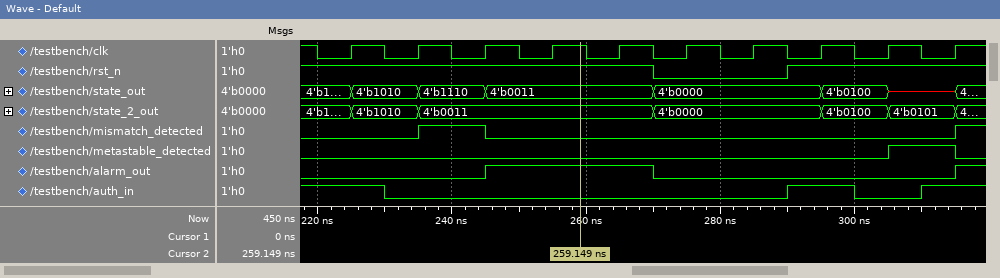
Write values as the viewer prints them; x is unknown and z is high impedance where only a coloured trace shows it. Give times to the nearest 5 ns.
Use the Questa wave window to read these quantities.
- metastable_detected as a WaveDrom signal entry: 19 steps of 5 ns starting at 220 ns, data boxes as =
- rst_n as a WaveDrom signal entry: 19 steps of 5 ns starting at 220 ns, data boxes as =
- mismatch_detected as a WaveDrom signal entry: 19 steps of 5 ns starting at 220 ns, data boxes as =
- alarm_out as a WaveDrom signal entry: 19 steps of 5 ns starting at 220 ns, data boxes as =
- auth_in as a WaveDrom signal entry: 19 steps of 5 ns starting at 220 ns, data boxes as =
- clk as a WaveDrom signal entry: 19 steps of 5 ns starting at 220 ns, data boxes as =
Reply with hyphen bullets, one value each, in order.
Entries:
- {name: 'metastable_detected', wave: '0................1.'}
- {name: 'rst_n', wave: '1.........0...1....'}
- {name: 'mismatch_detected', wave: '0..1.0.............'}
- {name: 'alarm_out', wave: '0....1....0........'}
- {name: 'auth_in', wave: '1.0...........1.0.1'}
- {name: 'clk', wave: '0101010101010101010'}
